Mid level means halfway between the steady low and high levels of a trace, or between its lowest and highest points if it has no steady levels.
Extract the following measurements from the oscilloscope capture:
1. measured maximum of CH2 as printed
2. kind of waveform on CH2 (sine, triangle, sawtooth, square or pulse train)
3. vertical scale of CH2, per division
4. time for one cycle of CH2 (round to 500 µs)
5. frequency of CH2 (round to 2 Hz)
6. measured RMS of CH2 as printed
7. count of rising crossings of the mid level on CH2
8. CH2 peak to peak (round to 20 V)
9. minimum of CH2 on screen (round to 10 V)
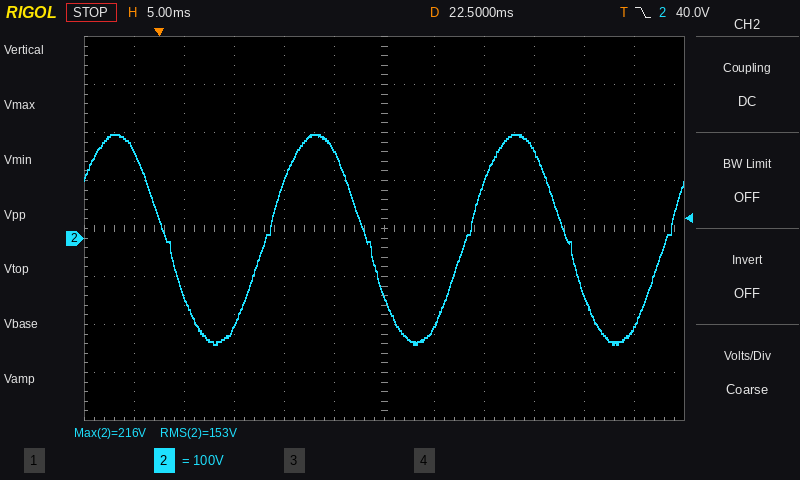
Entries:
216 V
sine
100 V
20.0 ms
50 Hz
153 V
3
440 V
-220 V
